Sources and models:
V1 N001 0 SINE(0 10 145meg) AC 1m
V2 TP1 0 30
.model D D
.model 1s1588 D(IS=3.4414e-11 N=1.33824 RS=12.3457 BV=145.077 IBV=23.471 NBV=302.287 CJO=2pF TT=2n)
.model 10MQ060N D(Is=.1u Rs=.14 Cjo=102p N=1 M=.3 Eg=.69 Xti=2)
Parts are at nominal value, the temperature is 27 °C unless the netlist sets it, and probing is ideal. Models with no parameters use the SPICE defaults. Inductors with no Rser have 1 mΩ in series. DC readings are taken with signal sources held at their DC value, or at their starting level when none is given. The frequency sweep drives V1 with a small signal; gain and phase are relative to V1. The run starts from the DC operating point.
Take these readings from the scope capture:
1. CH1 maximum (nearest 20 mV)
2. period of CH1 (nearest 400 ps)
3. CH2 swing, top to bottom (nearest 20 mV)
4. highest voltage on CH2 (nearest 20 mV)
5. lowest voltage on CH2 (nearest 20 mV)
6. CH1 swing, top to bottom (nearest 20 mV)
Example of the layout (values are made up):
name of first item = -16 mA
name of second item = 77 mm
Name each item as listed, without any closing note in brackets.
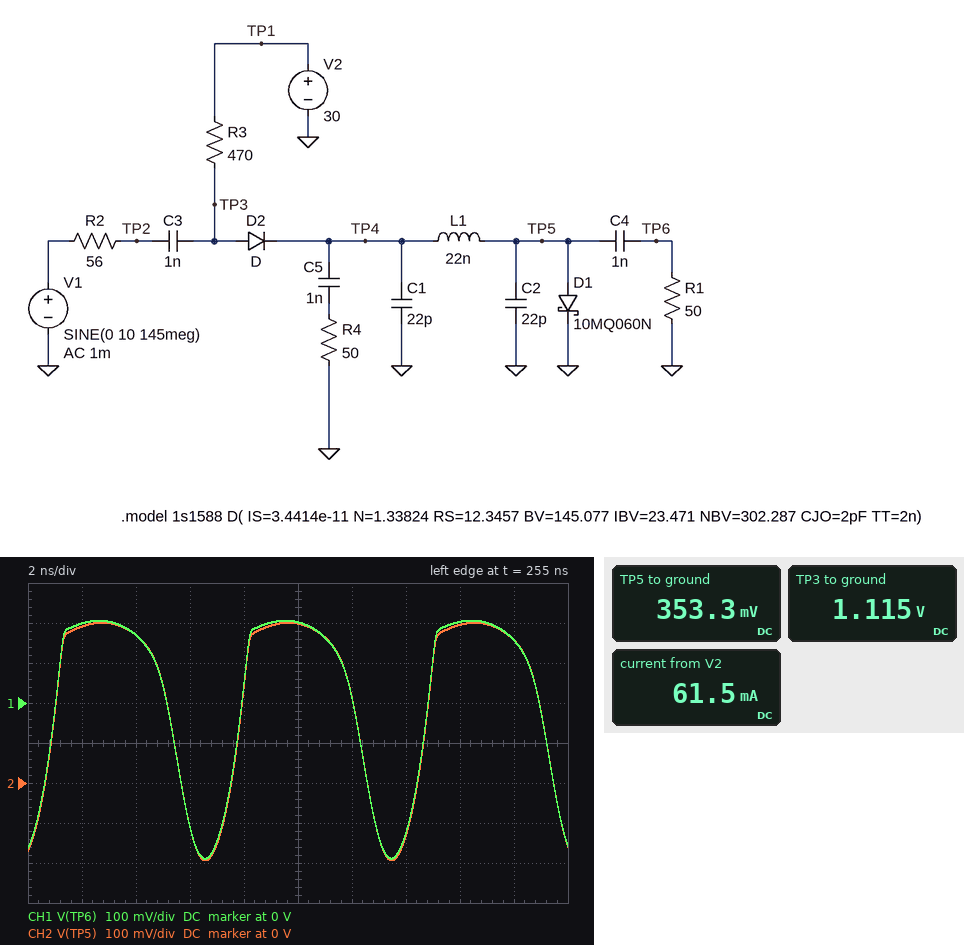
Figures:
CH1 maximum = 200 mV
period of CH1 = 6.8 ns
CH2 swing, top to bottom = 600 mV
highest voltage on CH2 = 400 mV
lowest voltage on CH2 = -200 mV
CH1 swing, top to bottom = 600 mV
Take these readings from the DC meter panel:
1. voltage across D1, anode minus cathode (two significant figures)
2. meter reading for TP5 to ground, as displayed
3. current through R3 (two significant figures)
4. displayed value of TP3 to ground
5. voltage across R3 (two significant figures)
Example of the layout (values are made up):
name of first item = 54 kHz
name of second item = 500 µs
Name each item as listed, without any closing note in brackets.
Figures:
voltage across D1, anode minus cathode = 350 mV
meter reading for TP5 to ground, as displayed = 353.3 mV
current through R3 = 61 mA
displayed value of TP3 to ground = 1.115 V
voltage across R3 = 29 V
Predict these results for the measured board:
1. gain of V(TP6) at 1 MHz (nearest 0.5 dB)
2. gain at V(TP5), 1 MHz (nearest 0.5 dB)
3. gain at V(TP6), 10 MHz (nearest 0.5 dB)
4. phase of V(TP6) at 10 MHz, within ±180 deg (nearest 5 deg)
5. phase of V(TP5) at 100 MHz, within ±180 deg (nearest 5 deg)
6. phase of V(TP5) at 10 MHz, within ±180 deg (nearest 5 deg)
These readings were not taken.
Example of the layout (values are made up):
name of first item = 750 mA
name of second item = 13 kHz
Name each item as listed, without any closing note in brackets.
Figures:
gain of V(TP6) at 1 MHz = -60.0 dB
gain at V(TP5), 1 MHz = -49.5 dB
gain at V(TP6), 10 MHz = -41.0 dB
phase of V(TP6) at 10 MHz, within ±180 deg = 30 deg
phase of V(TP5) at 100 MHz, within ±180 deg = -35 deg
phase of V(TP5) at 10 MHz, within ±180 deg = 10 deg
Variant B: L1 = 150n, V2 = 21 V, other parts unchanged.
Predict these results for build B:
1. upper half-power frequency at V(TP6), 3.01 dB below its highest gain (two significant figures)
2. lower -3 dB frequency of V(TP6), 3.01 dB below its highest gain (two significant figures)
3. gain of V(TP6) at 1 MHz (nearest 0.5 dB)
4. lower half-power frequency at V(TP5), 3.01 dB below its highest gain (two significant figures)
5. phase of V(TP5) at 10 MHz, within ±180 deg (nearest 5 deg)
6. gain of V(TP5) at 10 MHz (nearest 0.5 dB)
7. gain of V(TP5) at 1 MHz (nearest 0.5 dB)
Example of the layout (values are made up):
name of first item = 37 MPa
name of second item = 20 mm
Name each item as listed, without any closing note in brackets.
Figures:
upper half-power frequency at V(TP6), 3.01 dB below its highest gain = 34 MHz
lower -3 dB frequency of V(TP6), 3.01 dB below its highest gain = 3.9 MHz
gain of V(TP6) at 1 MHz = -57.5 dB
lower half-power frequency at V(TP5), 3.01 dB below its highest gain = 2.5 MHz
phase of V(TP5) at 10 MHz, within ±180 deg = -5 deg
gain of V(TP5) at 10 MHz = -38.0 dB
gain of V(TP5) at 1 MHz = -47.0 dB
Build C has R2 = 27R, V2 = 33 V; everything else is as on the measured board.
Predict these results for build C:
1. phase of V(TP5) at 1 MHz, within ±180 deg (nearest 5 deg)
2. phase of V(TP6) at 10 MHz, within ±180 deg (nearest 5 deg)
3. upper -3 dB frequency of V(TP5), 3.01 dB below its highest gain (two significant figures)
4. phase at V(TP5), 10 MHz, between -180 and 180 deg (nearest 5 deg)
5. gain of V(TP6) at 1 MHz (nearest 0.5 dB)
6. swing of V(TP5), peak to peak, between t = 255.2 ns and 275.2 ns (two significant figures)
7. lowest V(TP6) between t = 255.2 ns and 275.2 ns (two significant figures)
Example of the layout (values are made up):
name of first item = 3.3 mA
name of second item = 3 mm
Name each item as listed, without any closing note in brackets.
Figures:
phase of V(TP5) at 1 MHz, within ±180 deg = 80 deg
phase of V(TP6) at 10 MHz, within ±180 deg = 45 deg
upper -3 dB frequency of V(TP5), 3.01 dB below its highest gain = 170 MHz
phase at V(TP5), 10 MHz, between -180 and 180 deg = 25 deg
gain of V(TP6) at 1 MHz = -60.5 dB
swing of V(TP5), peak to peak, between t = 255.2 ns and 275.2 ns = 810 mV
lowest V(TP6) between t = 255.2 ns and 275.2 ns = -520 mV
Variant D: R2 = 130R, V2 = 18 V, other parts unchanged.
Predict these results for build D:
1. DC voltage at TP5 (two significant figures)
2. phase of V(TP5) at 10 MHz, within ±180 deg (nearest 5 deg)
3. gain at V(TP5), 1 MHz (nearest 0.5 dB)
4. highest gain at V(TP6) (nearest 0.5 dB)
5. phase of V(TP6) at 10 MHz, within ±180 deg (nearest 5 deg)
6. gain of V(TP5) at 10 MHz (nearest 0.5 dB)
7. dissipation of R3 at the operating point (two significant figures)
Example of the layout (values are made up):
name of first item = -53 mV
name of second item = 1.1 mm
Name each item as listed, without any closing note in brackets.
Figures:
DC voltage at TP5 = 340 mV
phase of V(TP5) at 10 MHz, within ±180 deg = 5 deg
gain at V(TP5), 1 MHz = -47.5 dB
highest gain at V(TP6) = -42.5 dB
phase of V(TP6) at 10 MHz, within ±180 deg = 20 deg
gain of V(TP5) at 10 MHz = -44.0 dB
dissipation of R3 at the operating point = 610 mW
